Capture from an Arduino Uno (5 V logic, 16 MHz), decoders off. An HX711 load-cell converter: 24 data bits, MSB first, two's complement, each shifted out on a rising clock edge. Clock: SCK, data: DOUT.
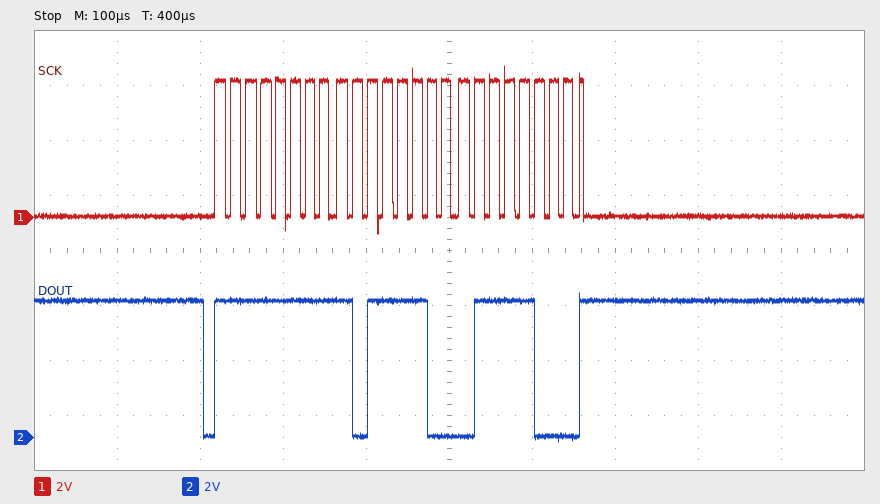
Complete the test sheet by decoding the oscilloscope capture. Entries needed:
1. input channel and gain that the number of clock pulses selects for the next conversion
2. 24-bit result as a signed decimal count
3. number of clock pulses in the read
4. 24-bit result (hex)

channel A, gain 128
-17288
25
0xFFBC78
